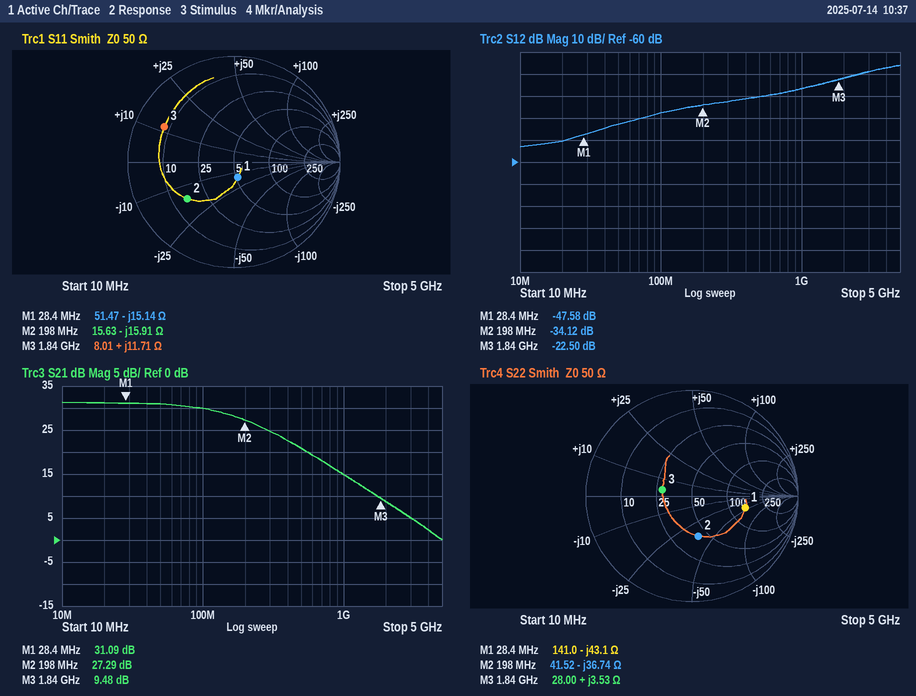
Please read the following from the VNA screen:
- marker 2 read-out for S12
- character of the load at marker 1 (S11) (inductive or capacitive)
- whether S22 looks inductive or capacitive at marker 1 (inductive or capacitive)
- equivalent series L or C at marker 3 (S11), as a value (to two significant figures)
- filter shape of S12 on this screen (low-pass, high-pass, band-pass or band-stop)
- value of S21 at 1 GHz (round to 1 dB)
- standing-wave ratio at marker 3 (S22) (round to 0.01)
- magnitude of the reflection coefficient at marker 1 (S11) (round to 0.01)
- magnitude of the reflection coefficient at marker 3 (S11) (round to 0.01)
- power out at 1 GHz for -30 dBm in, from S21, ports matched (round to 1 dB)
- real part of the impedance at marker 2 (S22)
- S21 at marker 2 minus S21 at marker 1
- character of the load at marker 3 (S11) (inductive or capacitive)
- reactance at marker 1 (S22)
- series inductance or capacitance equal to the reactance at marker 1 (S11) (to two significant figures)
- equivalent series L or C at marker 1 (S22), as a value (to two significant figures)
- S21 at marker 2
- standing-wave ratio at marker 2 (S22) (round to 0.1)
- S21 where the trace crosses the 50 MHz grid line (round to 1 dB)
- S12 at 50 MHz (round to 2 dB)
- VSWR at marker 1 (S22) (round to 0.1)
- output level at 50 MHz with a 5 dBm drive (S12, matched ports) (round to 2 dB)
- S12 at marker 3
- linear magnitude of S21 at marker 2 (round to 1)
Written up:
-34.12 dB
capacitive
capacitive
1.0 nH
high-pass
15 dB
1.80
0.15
0.74
-15 dBm
41.52 Ω
-3.80 dB
inductive
-43.1 Ω
370 pF
130 pF
27.29 dB
2.2
31 dB
-42 dB
3.1
-38 dBm
-22.50 dB
23
